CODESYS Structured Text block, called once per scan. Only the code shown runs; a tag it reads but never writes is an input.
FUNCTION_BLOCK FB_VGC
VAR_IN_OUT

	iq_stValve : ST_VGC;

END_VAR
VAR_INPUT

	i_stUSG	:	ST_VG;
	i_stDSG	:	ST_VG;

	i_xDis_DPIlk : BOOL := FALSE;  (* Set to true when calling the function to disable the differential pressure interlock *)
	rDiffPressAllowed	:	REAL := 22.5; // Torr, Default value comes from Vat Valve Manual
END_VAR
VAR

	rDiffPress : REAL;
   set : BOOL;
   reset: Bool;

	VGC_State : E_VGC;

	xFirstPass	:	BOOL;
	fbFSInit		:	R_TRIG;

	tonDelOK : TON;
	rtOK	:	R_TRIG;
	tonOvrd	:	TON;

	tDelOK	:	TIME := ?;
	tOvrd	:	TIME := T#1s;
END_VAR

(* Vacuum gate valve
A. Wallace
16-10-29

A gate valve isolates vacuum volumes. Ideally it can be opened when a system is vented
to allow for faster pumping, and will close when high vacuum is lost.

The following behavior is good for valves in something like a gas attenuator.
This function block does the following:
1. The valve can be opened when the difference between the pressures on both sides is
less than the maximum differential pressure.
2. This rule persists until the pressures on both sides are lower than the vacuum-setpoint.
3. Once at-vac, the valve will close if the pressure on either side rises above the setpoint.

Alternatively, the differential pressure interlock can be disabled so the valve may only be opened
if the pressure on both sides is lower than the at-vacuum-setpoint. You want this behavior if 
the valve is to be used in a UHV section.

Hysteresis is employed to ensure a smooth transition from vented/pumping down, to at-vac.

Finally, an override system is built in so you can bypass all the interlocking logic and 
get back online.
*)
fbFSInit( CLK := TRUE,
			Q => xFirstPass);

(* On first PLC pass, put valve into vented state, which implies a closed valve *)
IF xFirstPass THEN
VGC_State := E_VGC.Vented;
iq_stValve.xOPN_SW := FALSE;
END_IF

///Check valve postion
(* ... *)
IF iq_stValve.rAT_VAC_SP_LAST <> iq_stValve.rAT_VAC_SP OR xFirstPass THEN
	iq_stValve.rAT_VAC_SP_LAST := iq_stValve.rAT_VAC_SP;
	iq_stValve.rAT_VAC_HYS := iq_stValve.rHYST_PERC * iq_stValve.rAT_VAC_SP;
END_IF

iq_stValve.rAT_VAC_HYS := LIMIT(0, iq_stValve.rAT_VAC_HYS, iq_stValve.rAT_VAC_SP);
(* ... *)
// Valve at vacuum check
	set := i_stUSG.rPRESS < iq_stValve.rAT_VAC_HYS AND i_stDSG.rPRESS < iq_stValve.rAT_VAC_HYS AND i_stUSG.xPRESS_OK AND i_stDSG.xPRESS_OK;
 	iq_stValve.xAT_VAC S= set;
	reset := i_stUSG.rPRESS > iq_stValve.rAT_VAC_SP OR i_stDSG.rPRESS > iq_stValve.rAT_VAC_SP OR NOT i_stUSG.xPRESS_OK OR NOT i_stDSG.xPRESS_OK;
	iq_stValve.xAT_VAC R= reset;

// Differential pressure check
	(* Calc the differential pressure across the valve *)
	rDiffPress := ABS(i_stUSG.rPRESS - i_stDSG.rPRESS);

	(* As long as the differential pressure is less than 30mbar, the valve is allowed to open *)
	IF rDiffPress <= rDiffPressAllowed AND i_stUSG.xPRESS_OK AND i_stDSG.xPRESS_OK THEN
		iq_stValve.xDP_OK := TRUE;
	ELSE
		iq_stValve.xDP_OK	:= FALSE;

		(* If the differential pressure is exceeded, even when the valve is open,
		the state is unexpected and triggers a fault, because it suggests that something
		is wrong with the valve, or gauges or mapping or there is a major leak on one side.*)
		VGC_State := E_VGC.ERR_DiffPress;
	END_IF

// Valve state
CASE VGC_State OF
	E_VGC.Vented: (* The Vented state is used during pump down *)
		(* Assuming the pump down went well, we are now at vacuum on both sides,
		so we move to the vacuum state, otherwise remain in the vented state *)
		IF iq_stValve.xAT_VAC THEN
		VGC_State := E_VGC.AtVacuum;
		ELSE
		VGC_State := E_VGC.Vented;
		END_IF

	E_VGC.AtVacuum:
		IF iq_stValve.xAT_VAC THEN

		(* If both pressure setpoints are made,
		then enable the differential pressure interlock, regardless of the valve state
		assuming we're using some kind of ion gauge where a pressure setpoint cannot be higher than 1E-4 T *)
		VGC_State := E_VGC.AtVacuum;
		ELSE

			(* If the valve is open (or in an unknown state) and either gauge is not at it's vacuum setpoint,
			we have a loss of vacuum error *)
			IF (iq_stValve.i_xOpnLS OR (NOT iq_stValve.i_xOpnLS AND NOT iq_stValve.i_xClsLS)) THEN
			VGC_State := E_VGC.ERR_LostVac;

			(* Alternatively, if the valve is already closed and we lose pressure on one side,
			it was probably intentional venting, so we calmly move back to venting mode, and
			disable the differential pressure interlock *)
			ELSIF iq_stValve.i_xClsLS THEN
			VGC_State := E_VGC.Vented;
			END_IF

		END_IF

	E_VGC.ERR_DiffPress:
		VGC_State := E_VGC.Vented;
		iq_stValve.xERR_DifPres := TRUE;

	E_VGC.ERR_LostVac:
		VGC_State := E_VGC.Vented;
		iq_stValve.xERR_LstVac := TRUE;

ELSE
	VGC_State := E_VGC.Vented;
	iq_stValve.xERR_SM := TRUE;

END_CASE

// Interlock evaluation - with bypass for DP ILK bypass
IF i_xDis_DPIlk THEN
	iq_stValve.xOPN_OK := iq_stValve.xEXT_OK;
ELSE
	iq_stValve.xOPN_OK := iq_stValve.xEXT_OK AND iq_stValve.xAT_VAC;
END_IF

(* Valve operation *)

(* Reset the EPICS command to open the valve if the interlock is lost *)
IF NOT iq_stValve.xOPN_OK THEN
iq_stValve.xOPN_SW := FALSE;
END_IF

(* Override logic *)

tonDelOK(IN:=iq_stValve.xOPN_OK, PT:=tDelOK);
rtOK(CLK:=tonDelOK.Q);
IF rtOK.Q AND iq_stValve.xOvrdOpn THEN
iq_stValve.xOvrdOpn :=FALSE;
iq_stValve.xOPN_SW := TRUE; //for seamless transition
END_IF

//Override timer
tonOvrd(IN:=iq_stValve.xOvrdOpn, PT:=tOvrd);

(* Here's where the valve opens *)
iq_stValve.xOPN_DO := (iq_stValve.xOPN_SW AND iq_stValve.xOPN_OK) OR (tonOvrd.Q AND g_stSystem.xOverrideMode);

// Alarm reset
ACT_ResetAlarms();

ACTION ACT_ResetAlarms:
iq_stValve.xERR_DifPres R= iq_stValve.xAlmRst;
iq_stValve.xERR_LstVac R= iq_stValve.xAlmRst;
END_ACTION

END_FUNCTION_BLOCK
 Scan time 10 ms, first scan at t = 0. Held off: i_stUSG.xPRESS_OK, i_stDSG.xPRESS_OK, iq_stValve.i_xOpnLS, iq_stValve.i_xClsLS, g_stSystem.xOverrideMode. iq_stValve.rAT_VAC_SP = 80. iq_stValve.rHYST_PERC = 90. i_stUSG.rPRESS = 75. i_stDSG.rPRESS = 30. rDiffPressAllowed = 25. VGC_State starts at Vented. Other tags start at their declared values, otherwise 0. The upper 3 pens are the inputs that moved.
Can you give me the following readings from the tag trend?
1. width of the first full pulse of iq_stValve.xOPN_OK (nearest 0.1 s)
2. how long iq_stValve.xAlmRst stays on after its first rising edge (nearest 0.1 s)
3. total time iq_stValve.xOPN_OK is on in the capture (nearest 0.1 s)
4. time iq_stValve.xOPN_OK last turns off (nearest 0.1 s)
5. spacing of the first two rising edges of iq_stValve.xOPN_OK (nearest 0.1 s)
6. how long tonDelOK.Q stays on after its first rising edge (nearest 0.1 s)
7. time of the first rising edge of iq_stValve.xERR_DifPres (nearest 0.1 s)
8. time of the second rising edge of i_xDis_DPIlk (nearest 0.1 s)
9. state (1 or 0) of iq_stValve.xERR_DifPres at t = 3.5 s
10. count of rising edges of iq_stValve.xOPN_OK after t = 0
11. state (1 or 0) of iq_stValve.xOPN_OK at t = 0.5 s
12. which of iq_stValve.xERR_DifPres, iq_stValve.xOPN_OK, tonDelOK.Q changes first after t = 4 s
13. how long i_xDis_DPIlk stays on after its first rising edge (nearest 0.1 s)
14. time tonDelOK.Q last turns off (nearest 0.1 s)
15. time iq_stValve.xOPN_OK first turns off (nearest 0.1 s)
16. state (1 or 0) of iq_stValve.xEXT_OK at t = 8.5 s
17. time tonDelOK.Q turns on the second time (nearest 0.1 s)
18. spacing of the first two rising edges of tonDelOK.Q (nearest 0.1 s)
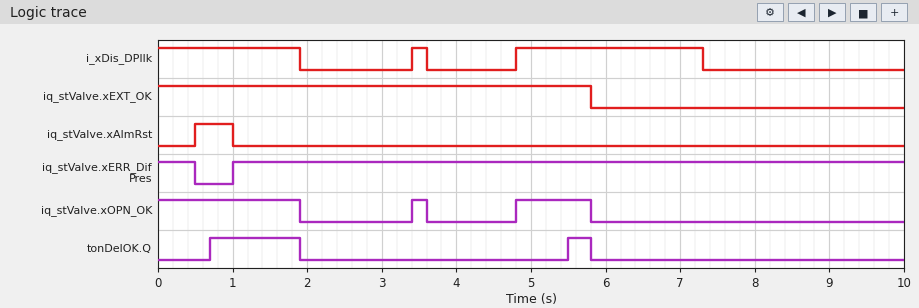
0.2 s
0.5 s
3.1 s
5.8 s
1.4 s
1.2 s
1.0 s
4.8 s
1
2
1
iq_stValve.xOPN_OK
0.2 s
5.8 s
1.9 s
0
5.5 s
4.8 s
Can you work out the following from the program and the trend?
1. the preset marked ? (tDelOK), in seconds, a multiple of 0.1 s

0.7 s
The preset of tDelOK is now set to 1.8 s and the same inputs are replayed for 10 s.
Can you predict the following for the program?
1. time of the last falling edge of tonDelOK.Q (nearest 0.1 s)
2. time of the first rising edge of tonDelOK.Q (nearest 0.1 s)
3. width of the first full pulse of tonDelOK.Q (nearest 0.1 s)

1.9 s
1.8 s
0.1 s
